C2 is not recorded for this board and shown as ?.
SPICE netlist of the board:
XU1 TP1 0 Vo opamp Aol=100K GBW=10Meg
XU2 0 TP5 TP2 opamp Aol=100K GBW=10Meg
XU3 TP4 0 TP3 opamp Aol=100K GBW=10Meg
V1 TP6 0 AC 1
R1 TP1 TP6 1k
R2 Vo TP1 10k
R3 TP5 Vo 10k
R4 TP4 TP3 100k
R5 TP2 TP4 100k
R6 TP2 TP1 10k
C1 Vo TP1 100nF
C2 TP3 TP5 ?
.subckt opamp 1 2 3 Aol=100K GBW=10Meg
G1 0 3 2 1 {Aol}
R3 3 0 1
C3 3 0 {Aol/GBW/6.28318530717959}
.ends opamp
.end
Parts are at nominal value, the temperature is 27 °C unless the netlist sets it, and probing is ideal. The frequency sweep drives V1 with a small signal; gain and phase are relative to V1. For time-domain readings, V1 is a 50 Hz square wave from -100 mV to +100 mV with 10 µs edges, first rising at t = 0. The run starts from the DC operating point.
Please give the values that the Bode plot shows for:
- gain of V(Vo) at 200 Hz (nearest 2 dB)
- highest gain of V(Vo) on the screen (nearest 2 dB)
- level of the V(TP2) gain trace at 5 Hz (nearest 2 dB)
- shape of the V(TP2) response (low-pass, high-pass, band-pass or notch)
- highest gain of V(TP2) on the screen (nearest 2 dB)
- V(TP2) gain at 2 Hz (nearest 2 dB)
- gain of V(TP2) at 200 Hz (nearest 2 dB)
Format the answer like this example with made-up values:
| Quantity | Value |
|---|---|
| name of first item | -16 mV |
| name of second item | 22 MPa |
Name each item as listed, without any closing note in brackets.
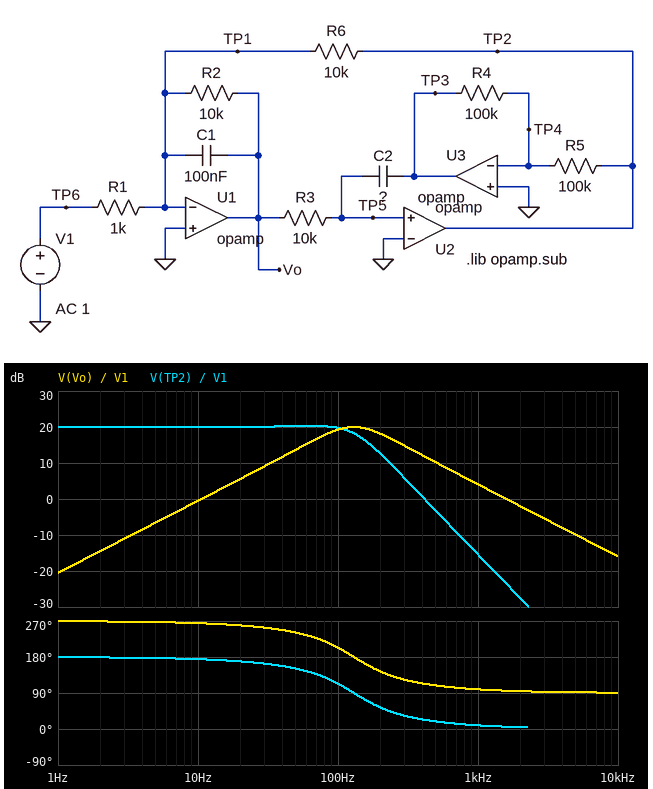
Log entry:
| Quantity | Value |
|---|---|
| gain of V(Vo) at 200 Hz | 18 dB |
| highest gain of V(Vo) on the screen | 20 dB |
| level of the V(TP2) gain trace at 5 Hz | 20 dB |
| shape of the V(TP2) response | low-pass |
| highest gain of V(TP2) on the screen | 20 dB |
| V(TP2) gain at 2 Hz | 20 dB |
| gain of V(TP2) at 200 Hz | 12 dB |
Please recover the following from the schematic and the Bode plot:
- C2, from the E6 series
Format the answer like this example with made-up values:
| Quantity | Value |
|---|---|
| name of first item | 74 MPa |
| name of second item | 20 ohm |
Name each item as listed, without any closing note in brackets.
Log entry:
| Quantity | Value |
|---|---|
| C2, from the E6 series | 150 nF |
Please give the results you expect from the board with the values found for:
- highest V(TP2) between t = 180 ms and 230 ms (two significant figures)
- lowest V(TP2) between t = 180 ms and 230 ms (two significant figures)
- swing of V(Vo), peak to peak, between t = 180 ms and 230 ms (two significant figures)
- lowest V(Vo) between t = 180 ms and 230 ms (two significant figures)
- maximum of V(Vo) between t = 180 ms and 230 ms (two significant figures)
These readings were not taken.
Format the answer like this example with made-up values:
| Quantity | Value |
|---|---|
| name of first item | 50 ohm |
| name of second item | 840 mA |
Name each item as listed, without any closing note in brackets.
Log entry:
| Quantity | Value |
|---|---|
| highest V(TP2) between t = 180 ms and 230 ms | 1.2 V |
| lowest V(TP2) between t = 180 ms and 230 ms | -1.2 V |
| swing of V(Vo), peak to peak, between t = 180 ms and 230 ms | 2.4 V |
| lowest V(Vo) between t = 180 ms and 230 ms | -1.2 V |
| maximum of V(Vo) between t = 180 ms and 230 ms | 1.2 V |
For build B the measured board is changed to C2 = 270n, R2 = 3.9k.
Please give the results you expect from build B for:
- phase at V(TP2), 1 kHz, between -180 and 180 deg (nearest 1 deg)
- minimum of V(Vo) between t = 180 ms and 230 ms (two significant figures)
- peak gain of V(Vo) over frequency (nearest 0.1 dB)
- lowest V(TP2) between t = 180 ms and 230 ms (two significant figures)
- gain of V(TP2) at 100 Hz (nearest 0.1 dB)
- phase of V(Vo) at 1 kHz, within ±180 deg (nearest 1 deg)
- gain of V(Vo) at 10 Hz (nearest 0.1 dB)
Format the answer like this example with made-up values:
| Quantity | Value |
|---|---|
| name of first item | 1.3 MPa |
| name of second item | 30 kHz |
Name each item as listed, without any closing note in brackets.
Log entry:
| Quantity | Value |
|---|---|
| phase at V(TP2), 1 kHz, between -180 and 180 deg | 22 deg |
| minimum of V(Vo) between t = 180 ms and 230 ms | -560 mV |
| peak gain of V(Vo) over frequency | 11.8 dB |
| lowest V(TP2) between t = 180 ms and 230 ms | -620 mV |
| gain of V(TP2) at 100 Hz | 7.2 dB |
| phase of V(Vo) at 1 kHz, within ±180 deg | 112 deg |
| gain of V(Vo) at 10 Hz | 3.9 dB |
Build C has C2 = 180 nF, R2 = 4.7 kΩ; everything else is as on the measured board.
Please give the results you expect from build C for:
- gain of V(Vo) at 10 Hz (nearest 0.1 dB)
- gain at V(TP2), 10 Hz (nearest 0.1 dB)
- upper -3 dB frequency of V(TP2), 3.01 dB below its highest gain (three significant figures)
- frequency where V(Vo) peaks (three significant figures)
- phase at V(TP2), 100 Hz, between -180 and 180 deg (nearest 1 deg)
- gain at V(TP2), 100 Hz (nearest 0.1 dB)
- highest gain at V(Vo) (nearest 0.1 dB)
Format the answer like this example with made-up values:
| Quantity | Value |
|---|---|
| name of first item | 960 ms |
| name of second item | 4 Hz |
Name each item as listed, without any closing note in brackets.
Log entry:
| Quantity | Value |
|---|---|
| gain of V(Vo) at 10 Hz | 0.9 dB |
| gain at V(TP2), 10 Hz | 19.8 dB |
| upper -3 dB frequency of V(TP2), 3.01 dB below its highest gain | 47.2 Hz |
| frequency where V(Vo) peaks | 119 Hz |
| phase at V(TP2), 100 Hz, between -180 and 180 deg | 97 deg |
| gain at V(TP2), 100 Hz | 12.3 dB |
| highest gain at V(Vo) | 13.4 dB |
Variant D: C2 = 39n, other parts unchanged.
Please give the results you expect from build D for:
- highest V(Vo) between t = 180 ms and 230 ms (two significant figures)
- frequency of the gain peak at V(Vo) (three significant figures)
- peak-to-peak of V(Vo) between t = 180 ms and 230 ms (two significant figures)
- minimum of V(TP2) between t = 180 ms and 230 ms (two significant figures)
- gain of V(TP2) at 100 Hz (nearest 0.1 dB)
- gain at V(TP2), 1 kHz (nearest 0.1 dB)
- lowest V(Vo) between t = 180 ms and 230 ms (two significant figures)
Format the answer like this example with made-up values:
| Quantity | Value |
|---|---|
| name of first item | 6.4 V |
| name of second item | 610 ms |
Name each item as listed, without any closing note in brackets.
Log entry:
| Quantity | Value |
|---|---|
| highest V(Vo) between t = 180 ms and 230 ms | 830 mV |
| frequency of the gain peak at V(Vo) | 255 Hz |
| peak-to-peak of V(Vo) between t = 180 ms and 230 ms | 1.7 V |
| minimum of V(TP2) between t = 180 ms and 230 ms | -1.7 V |
| gain of V(TP2) at 100 Hz | 21.1 dB |
| gain at V(TP2), 1 kHz | -3.3 dB |
| lowest V(Vo) between t = 180 ms and 230 ms | -830 mV |
